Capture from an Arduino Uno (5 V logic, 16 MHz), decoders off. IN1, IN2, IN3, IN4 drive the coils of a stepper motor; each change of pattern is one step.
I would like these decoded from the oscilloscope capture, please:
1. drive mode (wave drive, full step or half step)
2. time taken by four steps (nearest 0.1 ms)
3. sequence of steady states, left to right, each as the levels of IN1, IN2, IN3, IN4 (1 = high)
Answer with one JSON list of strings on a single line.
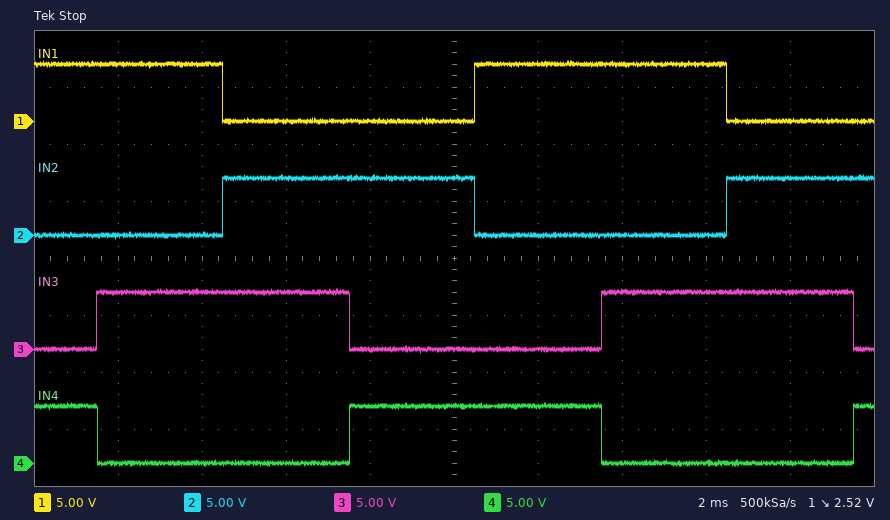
["full step", "12.0 ms", "1001 1010 0110 0101 1001 1010 0110 0101"]
